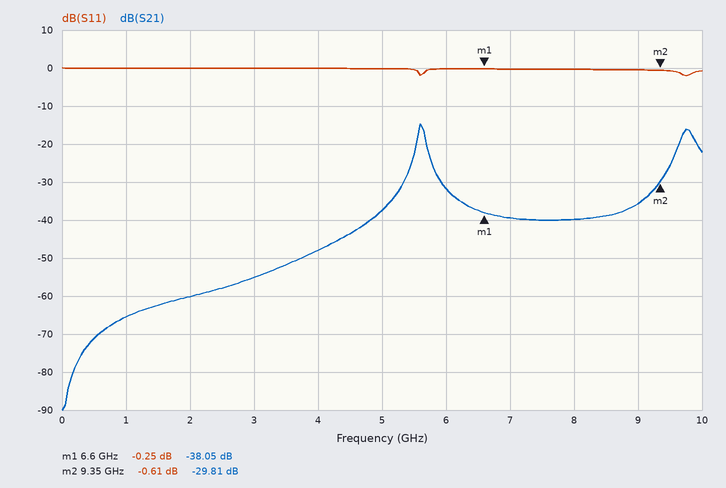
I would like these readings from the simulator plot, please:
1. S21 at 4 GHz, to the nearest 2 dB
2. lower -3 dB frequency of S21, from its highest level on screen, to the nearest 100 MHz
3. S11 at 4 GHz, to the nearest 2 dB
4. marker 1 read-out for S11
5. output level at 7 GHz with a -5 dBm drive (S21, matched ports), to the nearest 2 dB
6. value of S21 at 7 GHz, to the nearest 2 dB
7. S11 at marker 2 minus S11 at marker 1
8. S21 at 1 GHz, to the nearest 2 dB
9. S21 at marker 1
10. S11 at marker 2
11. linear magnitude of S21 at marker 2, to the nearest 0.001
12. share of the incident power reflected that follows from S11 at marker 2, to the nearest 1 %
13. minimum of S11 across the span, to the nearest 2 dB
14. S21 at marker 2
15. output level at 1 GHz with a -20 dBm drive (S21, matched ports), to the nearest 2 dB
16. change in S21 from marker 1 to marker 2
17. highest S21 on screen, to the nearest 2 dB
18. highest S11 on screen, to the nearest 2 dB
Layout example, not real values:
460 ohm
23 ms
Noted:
-48 dB
5.6 GHz
0 dB
-0.25 dB
-44 dBm
-40 dB
-0.36 dB
-66 dB
-38.05 dB
-0.61 dB
0.032
87 %
-2 dB
-29.81 dB
-86 dBm
8.24 dB
-14 dB
0 dB
